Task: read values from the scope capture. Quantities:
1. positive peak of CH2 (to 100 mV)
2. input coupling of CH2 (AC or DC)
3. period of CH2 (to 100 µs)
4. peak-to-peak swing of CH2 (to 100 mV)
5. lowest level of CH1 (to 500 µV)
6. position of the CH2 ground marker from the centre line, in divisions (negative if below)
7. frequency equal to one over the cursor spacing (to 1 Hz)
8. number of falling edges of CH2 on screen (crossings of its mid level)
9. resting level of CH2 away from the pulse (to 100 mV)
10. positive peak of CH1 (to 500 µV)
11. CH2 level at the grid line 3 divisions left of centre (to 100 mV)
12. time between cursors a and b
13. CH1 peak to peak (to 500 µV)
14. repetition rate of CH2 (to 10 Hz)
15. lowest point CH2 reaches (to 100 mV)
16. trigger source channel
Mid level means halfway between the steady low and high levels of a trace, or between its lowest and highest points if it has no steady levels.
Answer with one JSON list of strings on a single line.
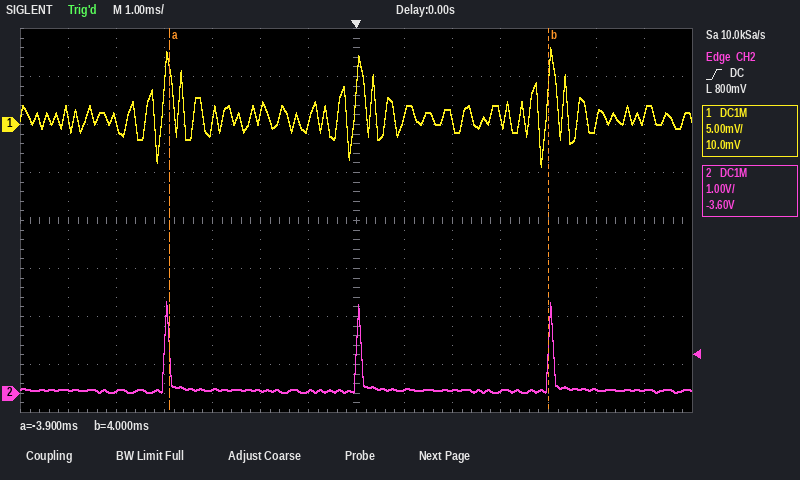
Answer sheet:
["1.9 V", "DC", "4.0 ms", "1.9 V", "-4.5 mV", "-3.6 div", "127 Hz", "3", "100 mV", "8.0 mV", "100 mV", "7.9 ms", "12.5 mV", "250 Hz", "0.0 V", "CH2"]
